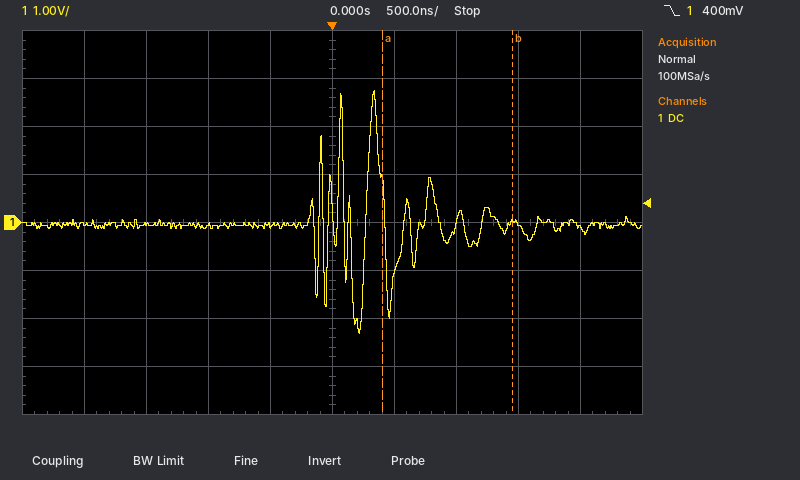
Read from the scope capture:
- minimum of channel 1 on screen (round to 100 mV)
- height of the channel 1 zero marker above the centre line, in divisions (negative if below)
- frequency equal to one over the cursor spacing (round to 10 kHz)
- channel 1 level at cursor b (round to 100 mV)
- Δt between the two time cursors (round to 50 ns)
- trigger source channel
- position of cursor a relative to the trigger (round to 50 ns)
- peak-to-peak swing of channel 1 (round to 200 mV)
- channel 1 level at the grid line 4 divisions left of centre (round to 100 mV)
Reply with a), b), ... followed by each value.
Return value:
a) -2.3 V
b) 0.0 div
c) 950 kHz
d) 0.0 V
e) 1.05 µs
f) channel 1
g) +400 ns
h) 5.0 V
i) 0.0 V
